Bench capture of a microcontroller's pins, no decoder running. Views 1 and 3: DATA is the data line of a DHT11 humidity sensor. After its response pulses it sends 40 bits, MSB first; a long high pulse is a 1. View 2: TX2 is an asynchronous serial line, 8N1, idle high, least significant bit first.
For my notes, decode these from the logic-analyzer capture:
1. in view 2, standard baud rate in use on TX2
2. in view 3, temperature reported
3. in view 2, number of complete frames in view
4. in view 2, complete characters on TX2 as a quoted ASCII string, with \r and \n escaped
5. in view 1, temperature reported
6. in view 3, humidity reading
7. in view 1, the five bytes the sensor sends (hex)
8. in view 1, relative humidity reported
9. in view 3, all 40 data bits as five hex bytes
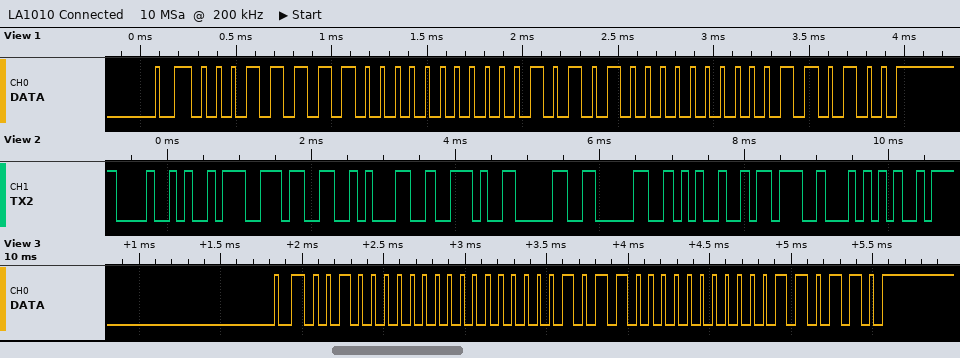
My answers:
9600 baud
22.0 °C
10
"H:31.00%;T"
21.0 °C
32 %
1F 00 15 00 34
31 %
20 00 16 00 36
